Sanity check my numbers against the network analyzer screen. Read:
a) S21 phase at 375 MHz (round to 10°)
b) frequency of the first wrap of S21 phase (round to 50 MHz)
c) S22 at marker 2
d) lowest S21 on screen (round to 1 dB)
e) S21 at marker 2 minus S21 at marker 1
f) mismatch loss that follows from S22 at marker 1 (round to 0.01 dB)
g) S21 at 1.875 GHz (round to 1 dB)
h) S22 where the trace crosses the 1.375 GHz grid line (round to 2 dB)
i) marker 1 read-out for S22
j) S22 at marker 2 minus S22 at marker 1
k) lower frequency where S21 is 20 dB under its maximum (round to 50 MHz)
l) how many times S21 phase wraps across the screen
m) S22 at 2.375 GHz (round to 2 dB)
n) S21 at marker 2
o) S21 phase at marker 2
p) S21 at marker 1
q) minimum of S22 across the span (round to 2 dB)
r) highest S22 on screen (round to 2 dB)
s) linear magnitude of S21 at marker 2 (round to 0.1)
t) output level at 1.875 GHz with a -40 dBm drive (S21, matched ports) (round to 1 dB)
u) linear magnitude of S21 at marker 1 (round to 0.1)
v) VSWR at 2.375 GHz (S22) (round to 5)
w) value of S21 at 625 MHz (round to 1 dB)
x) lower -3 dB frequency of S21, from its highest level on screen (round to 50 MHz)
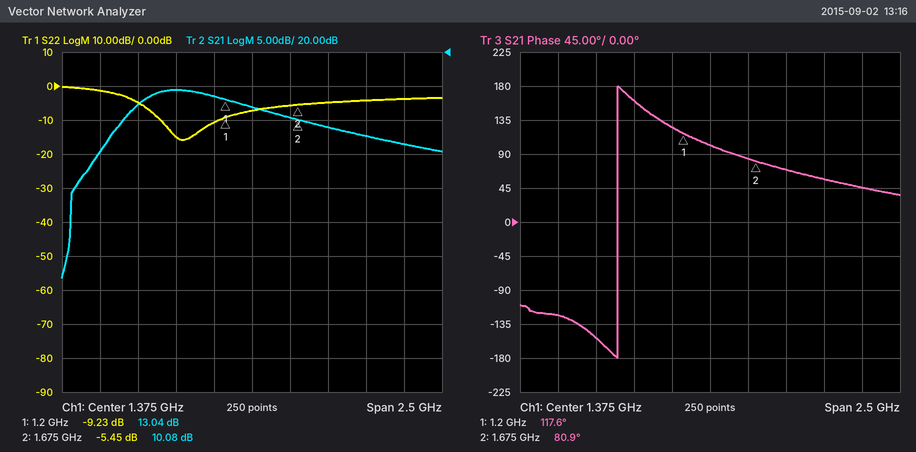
-120°
750 MHz
-5.45 dB
-13 dB
-2.96 dB
0.55 dB
9 dB
-8 dB
-9.23 dB
3.78 dB
200 MHz
1
-4 dB
10.08 dB
80.9°
13.04 dB
-16 dB
0 dB
3.2
-31 dBm
4.5
5
12 dB
600 MHz
